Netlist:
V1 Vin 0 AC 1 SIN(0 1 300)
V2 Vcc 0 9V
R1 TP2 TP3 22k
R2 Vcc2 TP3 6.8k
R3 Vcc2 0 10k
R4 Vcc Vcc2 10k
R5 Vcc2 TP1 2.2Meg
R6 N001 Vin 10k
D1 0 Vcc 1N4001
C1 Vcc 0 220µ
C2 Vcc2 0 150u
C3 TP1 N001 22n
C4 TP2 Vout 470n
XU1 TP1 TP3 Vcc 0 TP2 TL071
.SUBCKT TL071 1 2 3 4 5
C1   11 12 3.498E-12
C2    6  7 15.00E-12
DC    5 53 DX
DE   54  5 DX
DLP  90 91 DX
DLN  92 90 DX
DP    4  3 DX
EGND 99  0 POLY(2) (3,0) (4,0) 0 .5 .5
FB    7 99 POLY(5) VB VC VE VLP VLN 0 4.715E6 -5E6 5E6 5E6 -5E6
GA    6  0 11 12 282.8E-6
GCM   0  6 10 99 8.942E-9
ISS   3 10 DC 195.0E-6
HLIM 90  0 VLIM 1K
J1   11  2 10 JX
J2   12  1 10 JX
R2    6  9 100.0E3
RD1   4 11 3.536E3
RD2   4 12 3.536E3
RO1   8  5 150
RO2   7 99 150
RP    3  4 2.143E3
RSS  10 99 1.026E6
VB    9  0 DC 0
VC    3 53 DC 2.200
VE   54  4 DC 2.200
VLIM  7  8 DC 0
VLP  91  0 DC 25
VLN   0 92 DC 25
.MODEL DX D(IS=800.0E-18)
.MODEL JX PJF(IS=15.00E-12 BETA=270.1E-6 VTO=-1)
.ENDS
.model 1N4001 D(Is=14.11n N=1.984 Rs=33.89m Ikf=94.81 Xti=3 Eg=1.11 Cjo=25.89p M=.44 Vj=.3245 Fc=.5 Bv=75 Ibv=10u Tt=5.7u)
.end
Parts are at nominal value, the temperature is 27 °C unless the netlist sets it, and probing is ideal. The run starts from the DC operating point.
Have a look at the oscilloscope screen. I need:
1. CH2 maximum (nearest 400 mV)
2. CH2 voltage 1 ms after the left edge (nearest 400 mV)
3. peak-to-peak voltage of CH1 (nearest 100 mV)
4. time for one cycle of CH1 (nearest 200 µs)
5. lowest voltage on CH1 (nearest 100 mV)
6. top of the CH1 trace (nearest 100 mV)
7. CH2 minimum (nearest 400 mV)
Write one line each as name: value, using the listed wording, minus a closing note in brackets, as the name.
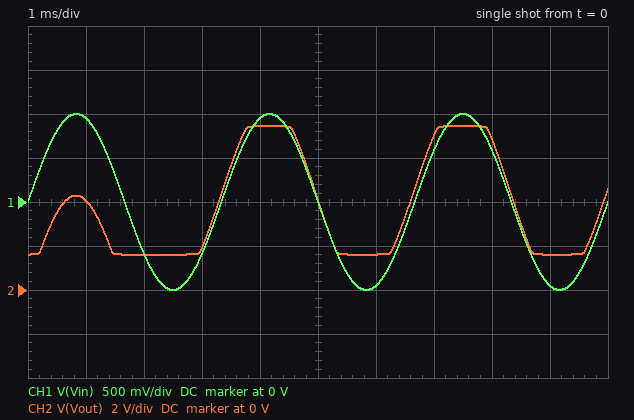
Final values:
CH2 maximum: 7.6 V
CH2 voltage 1 ms after the left edge: 4.0 V
peak-to-peak voltage of CH1: 2.0 V
time for one cycle of CH1: 3.4 ms
lowest voltage on CH1: -1.0 V
top of the CH1 trace: 1.0 V
CH2 minimum: 1.6 V
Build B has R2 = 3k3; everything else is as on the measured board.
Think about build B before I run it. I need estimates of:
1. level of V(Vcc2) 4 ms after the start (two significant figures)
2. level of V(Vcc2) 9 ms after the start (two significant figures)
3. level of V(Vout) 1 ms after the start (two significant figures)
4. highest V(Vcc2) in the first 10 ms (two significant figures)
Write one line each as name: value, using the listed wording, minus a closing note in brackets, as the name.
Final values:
level of V(Vcc2) 4 ms after the start: 29 mV
level of V(Vcc2) 9 ms after the start: 66 mV
level of V(Vout) 1 ms after the start: 7.3 V
highest V(Vcc2) in the first 10 ms: 72 mV
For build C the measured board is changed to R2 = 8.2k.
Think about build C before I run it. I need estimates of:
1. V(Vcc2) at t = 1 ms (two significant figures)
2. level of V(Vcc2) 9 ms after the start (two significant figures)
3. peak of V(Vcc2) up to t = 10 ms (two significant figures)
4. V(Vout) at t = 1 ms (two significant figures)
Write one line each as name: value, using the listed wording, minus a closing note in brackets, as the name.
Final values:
V(Vcc2) at t = 1 ms: 6.7 mV
level of V(Vcc2) 9 ms after the start: 61 mV
peak of V(Vcc2) up to t = 10 ms: 67 mV
V(Vout) at t = 1 ms: 3.5 V
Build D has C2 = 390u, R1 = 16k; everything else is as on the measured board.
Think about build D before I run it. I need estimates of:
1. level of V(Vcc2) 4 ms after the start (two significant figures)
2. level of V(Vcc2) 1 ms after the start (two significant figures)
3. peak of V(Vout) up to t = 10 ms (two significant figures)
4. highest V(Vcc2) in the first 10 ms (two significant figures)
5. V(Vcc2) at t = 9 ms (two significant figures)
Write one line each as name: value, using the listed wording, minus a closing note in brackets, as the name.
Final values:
level of V(Vcc2) 4 ms after the start: 10 mV
level of V(Vcc2) 1 ms after the start: 2.6 mV
peak of V(Vout) up to t = 10 ms: 7.0 V
highest V(Vcc2) in the first 10 ms: 27 mV
V(Vcc2) at t = 9 ms: 24 mV
